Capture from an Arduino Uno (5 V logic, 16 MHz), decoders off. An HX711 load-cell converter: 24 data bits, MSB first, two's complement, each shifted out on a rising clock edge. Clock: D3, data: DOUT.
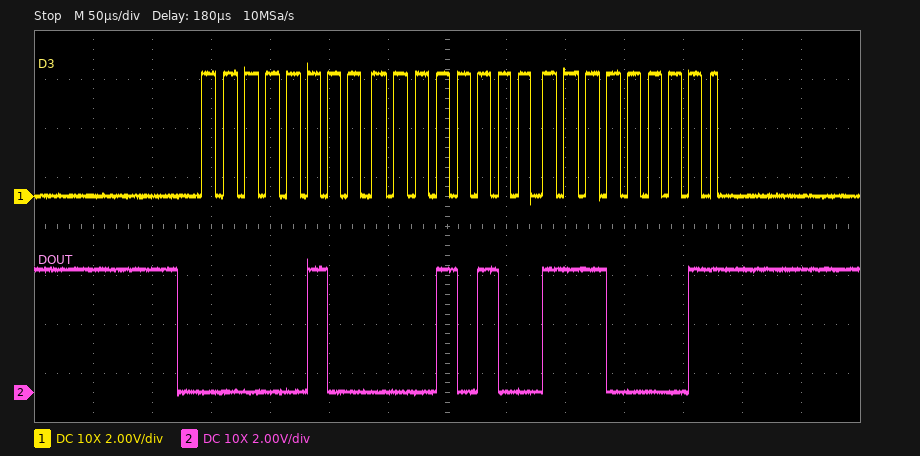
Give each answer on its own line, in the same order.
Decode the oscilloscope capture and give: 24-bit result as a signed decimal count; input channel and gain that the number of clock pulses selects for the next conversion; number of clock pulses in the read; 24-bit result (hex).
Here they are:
267489
channel A, gain 128
25
0x0414E1
